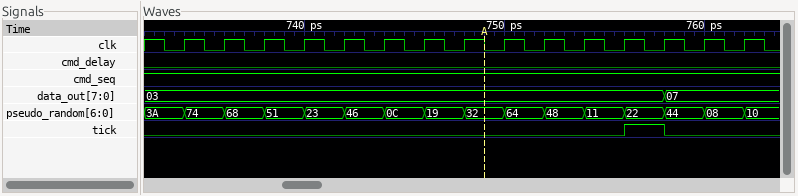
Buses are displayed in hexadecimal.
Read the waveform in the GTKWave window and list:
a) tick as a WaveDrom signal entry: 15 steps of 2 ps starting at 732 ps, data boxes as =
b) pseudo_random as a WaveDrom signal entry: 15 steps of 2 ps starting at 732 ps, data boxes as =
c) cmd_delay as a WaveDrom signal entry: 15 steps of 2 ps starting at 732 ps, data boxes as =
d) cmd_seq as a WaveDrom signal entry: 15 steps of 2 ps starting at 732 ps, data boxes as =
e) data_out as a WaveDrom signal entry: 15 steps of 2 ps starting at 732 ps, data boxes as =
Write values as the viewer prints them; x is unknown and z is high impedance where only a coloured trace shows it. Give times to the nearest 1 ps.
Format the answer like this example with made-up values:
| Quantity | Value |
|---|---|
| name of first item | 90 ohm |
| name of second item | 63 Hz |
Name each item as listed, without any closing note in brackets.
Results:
| Quantity | Value |
|---|---|
| tick as a WaveDrom signal entry: 15 steps of 2 ps starting at 732 ps, data boxes as = | {name: 'tick', wave: '0...........10.'} |
| pseudo_random as a WaveDrom signal entry: 15 steps of 2 ps starting at 732 ps, data boxes as = | {name: 'pseudo_random', wave: '===============', data: '3A 74 68 51 23 46 0C 19 32 64 48 11 22 44 08'} |
| cmd_delay as a WaveDrom signal entry: 15 steps of 2 ps starting at 732 ps, data boxes as = | {name: 'cmd_delay', wave: '0..............'} |
| cmd_seq as a WaveDrom signal entry: 15 steps of 2 ps starting at 732 ps, data boxes as = | {name: 'cmd_seq', wave: '1..............'} |
| data_out as a WaveDrom signal entry: 15 steps of 2 ps starting at 732 ps, data boxes as = | {name: 'data_out', wave: '=............=.', data: '03 07'} |
